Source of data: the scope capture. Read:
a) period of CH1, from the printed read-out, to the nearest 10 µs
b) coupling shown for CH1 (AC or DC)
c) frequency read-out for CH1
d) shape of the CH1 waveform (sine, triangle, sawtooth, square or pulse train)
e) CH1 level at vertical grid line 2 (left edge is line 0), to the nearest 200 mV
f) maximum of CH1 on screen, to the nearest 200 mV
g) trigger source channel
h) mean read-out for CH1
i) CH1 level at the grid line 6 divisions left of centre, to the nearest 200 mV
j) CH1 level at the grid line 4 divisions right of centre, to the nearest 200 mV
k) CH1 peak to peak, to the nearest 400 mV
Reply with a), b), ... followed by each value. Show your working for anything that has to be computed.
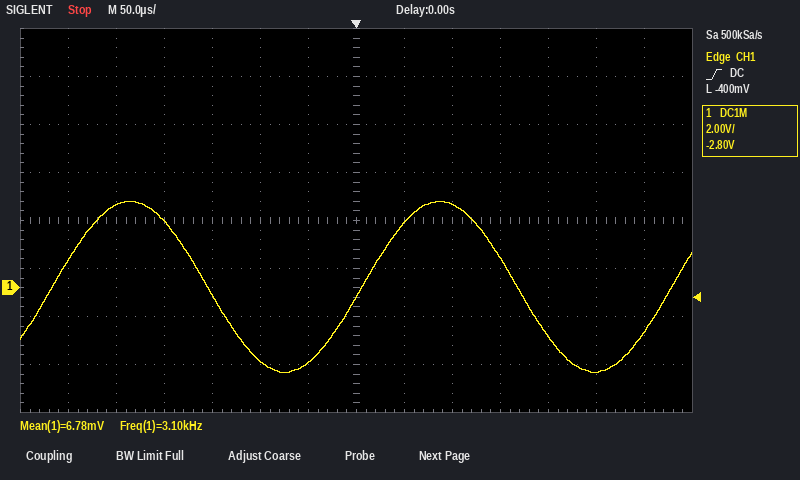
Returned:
a) 1 / 3.10 kHz ≈ 323 µs, so 320 µs to the nearest 10 µs
b) DC
c) 3.10 kHz
d) sine
e) 3.4 V
f) 3.6 V
g) CH1
h) 6.78 mV
i) 1.2 V
j) -2.0 V
k) 7.2 V
